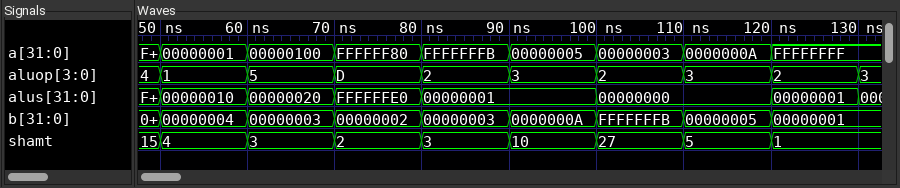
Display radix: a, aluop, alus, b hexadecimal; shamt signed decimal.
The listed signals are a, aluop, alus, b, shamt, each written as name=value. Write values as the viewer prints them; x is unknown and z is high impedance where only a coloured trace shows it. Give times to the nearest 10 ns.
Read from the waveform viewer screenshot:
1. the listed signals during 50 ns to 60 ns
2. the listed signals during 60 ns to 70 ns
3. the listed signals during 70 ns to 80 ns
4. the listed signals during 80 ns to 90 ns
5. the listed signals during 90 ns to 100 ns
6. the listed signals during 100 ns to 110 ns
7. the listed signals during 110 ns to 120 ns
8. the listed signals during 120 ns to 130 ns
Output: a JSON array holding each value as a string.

["a=00000001, aluop=1, alus=00000010, b=00000004, shamt=4", "a=00000100, aluop=5, alus=00000020, b=00000003, shamt=3", "a=FFFFFF80, aluop=D, alus=FFFFFFE0, b=00000002, shamt=2", "a=FFFFFFFB, aluop=2, alus=00000001, b=00000003, shamt=3", "a=00000005, aluop=3, alus=00000001, b=0000000A, shamt=10", "a=00000003, aluop=2, alus=00000000, b=FFFFFFFB, shamt=27", "a=0000000A, aluop=3, alus=00000000, b=00000005, shamt=5", "a=FFFFFFFF, aluop=2, alus=00000001, b=00000001, shamt=1"]
